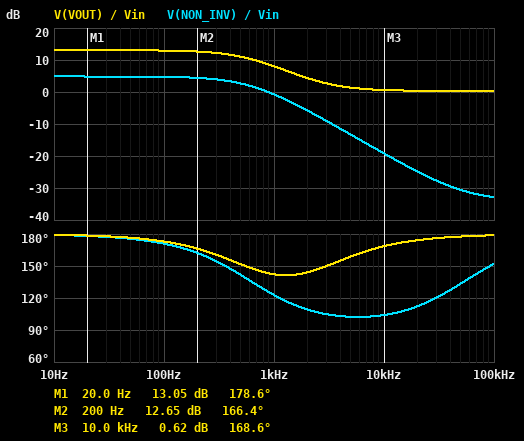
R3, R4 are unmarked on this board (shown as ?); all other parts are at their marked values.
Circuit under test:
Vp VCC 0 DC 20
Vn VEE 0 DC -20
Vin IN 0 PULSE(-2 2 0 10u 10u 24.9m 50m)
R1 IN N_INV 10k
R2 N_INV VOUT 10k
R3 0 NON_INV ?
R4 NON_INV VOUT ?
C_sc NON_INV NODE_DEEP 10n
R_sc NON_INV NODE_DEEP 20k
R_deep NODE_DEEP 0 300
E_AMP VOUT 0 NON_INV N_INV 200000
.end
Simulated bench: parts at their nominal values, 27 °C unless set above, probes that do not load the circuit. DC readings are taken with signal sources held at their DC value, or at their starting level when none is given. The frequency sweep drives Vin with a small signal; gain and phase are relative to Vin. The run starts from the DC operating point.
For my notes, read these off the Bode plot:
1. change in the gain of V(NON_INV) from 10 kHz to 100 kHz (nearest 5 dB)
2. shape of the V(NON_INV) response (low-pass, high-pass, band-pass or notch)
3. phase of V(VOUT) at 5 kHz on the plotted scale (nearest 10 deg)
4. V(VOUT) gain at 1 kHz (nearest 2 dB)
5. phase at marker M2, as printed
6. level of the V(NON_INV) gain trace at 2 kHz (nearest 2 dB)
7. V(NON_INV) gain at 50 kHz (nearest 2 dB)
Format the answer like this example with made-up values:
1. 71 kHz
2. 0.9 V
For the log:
1. -15 dB
2. low-pass
3. 160 deg
4. 8 dB
5. 166.4 deg
6. -6 dB
7. -30 dB
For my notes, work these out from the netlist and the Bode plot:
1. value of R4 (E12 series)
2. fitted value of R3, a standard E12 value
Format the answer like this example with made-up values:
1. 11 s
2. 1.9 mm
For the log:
1. 15 kΩ
2. 18 kΩ
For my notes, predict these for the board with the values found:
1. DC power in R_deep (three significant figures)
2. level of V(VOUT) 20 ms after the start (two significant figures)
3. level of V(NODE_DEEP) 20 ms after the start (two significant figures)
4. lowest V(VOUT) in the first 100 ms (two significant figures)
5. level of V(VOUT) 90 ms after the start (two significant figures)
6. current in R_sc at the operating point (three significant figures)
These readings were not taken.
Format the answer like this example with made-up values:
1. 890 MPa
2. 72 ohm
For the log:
1. 8.89 µW
2. -9.0 V
3. -52 mV
4. -9.0 V
5. 9.0 V
6. 172 µA
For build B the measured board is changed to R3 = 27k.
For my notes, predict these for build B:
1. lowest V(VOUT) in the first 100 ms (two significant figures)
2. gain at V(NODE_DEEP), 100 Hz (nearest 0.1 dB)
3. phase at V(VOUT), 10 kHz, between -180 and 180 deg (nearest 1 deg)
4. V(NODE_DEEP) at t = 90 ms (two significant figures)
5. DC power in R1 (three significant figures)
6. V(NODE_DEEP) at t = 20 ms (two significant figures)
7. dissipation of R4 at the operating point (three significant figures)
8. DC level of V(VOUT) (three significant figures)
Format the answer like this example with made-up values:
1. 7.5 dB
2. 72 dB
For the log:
1. -16 V
2. -26.3 dB
3. 168 deg
4. 100 mV
5. 7.73 mW
6. -100 mV
7. 5.15 mW
8. 15.6 V
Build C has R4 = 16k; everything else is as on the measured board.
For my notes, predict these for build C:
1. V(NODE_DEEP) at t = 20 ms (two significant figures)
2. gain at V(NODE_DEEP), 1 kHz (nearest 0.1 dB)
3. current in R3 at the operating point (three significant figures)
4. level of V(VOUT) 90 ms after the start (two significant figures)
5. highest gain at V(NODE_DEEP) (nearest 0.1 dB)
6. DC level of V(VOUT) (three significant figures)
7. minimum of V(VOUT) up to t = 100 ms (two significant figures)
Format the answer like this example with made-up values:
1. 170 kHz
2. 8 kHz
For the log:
1. -44 mV
2. -34.1 dB
3. 164 µA
4. 7.9 V
5. -33.2 dB
6. 7.91 V
7. -7.9 V
